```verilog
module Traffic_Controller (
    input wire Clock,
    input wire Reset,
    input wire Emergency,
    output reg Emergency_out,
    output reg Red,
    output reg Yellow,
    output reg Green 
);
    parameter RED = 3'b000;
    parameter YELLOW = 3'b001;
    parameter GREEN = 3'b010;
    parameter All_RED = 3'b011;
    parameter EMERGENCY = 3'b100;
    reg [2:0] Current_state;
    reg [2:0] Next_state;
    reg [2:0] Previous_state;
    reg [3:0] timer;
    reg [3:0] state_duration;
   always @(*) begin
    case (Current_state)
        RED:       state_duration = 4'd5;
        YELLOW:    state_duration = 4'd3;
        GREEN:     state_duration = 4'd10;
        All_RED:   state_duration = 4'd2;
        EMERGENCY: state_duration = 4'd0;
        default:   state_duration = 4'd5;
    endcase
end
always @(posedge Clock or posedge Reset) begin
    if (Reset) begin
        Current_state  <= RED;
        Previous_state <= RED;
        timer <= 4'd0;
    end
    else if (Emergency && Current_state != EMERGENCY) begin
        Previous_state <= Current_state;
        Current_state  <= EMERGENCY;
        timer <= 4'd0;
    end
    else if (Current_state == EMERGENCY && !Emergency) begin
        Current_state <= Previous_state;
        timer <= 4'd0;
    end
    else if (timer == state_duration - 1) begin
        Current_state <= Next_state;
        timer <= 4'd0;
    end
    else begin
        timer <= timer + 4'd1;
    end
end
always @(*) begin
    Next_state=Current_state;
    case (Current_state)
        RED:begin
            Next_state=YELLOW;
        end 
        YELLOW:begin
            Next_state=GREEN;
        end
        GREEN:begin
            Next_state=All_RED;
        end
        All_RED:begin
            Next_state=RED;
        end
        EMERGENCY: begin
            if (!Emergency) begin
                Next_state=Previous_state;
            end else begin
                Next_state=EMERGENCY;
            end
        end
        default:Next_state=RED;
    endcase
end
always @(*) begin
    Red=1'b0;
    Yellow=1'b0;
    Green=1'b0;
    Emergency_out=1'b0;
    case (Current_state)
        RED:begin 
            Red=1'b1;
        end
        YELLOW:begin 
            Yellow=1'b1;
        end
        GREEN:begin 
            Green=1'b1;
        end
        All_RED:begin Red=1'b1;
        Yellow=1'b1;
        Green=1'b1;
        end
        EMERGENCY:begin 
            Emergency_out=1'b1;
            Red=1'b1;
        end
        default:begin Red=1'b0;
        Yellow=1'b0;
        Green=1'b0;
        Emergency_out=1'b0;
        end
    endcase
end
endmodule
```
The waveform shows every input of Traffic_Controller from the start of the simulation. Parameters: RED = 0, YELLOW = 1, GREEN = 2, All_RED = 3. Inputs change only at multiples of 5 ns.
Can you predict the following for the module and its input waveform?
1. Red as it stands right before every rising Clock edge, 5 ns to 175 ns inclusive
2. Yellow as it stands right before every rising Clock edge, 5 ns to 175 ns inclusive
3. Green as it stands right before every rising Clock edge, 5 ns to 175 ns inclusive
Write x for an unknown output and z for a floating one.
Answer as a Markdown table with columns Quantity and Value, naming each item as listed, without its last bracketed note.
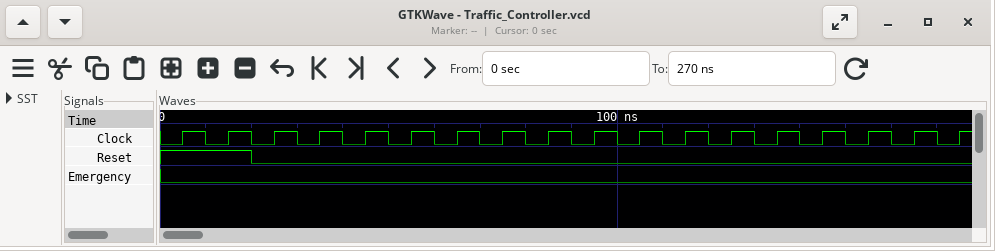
| Quantity | Value |
|---|---|
| Red as it stands right before every rising Clock edge, 5 ns to 175 ns inclusive | 1 1 1 1 1 1 1 0 0 0 0 0 0 0 0 0 0 0 |
| Yellow as it stands right before every rising Clock edge, 5 ns to 175 ns inclusive | 0 0 0 0 0 0 0 1 1 1 0 0 0 0 0 0 0 0 |
| Green as it stands right before every rising Clock edge, 5 ns to 175 ns inclusive | 0 0 0 0 0 0 0 0 0 0 1 1 1 1 1 1 1 1 |
